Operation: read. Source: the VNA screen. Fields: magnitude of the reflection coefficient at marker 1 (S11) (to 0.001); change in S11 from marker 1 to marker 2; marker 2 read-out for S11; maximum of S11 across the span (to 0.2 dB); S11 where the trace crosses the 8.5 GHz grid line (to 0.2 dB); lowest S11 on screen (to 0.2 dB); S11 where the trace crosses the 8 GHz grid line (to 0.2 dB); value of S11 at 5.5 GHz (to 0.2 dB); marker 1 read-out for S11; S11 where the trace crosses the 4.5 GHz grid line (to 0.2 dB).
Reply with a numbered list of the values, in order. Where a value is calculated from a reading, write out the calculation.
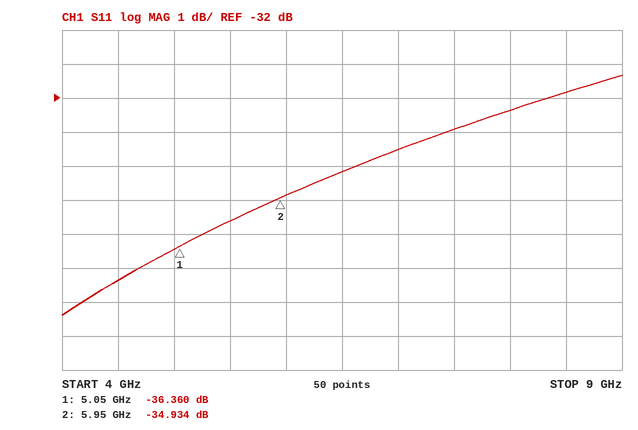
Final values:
1. 10^(-36.36/20) ≈ 0.015
2. -34.934 − (-36.36) = 1.426 dB
3. -34.934 dB
4. -31.4 dB
5. -31.8 dB
6. -38.4 dB
7. -32.4 dB
8. -35.6 dB
9. -36.360 dB
10. -37.4 dB
